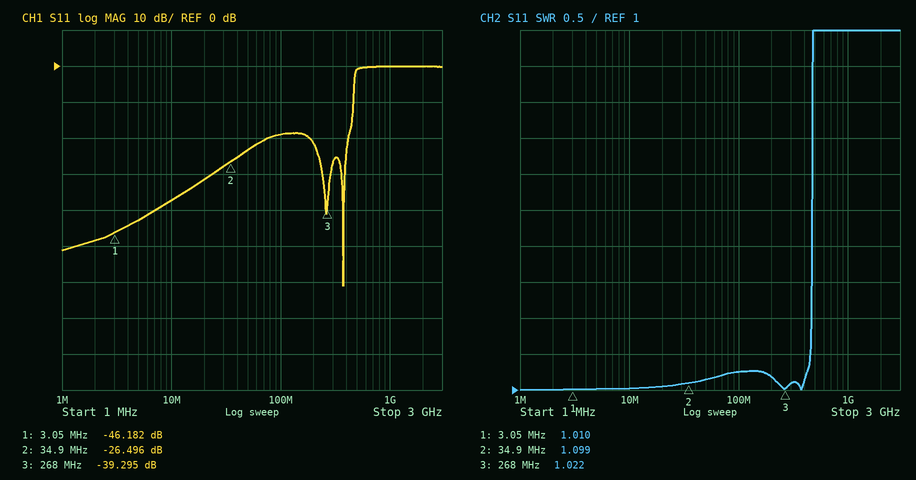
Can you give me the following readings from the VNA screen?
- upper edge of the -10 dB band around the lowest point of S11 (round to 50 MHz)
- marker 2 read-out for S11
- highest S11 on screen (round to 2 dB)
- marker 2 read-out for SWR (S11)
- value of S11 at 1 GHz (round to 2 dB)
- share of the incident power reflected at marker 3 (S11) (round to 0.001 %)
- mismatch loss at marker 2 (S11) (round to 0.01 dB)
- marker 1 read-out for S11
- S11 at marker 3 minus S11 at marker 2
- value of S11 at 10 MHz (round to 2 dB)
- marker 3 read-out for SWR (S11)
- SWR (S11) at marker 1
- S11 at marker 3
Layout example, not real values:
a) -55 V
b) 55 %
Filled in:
a) 450 MHz
b) -26.496 dB
c) 0 dB
d) 1.099
e) 0 dB
f) 0.012 %
g) 0.01 dB
h) -46.182 dB
i) -12.799 dB
j) -38 dB
k) 1.022
l) 1.010
m) -39.295 dB
